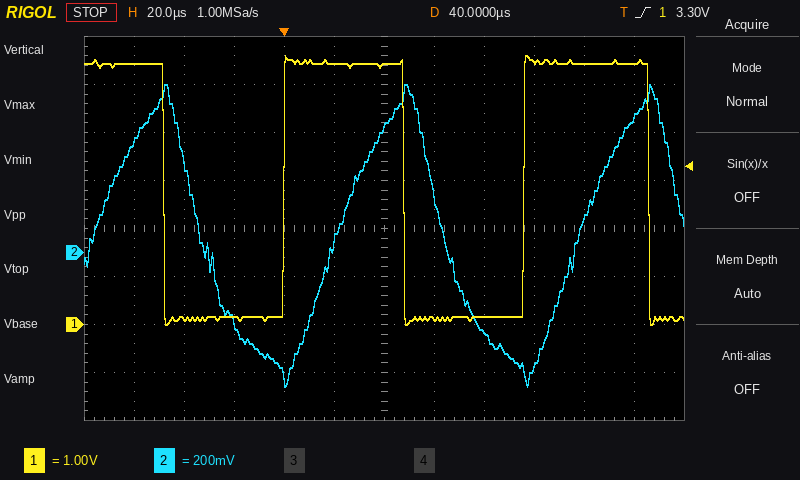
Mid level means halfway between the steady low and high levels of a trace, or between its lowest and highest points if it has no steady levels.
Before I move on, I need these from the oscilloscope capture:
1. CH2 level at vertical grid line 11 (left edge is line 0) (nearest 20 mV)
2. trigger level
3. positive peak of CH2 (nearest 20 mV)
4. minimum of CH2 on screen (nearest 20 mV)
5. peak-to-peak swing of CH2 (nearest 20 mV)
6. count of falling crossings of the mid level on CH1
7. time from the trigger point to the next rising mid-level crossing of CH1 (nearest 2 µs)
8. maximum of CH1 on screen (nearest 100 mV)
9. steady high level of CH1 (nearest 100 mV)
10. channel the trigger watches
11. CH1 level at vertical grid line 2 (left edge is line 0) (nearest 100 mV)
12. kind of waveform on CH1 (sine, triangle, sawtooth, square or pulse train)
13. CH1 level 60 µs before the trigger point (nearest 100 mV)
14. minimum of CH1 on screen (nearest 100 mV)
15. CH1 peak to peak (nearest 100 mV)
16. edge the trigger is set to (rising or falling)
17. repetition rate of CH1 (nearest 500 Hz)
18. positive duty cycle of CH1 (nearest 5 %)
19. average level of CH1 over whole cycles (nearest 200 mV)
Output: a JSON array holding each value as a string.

["560 mV", "3.30 V", "700 mV", "-560 mV", "1.26 V", "3", "96 µs", "5.6 V", "5.4 V", "CH1", "100 mV", "square", "5.4 V", "0.0 V", "5.6 V", "rising", "10.5 kHz", "50 %", "2.8 V"]
